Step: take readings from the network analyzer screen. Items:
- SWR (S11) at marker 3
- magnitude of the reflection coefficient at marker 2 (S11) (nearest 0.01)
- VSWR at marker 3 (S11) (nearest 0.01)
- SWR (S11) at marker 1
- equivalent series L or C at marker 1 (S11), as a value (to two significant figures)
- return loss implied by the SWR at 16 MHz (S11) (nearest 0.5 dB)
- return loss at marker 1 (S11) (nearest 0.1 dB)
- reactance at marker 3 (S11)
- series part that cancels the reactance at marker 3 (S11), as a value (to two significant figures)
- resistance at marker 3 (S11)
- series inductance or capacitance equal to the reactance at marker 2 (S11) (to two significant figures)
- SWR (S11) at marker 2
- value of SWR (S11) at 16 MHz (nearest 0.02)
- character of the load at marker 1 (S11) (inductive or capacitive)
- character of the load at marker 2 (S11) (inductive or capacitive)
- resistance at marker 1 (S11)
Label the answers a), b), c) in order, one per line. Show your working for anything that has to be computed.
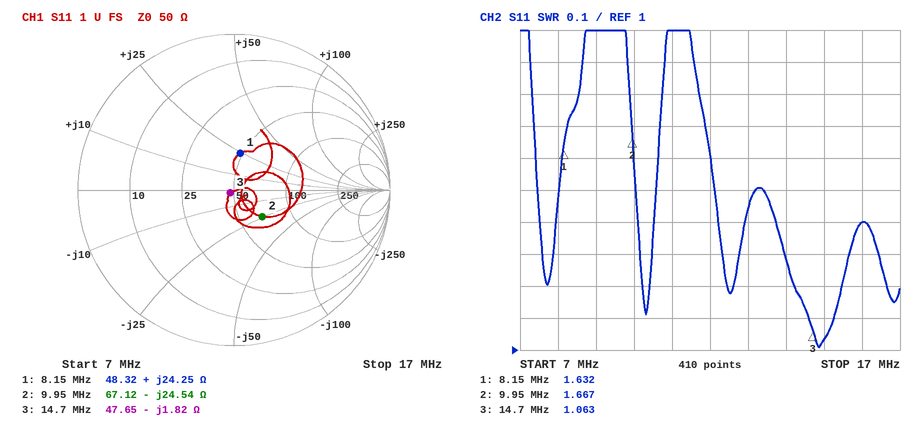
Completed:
a) 1.063
b) 0.25
c) 1.06
d) 1.632
e) L = 24.25 Ω/(2π × 8.15 MHz) ≈ 474 nH, so 470 nH to two significant figures
f) −20 log10((1.4 − 1)/(1.4 + 1)) ≈ 15.6 dB, so 15.5 dB to the nearest 0.5 dB
g) 12.4 dB
h) -1.82 Ω
i) L = 1.82 Ω/(2π × 14.7 MHz) ≈ 20 nH
j) 47.65 Ω
k) C = 1/(2π × 9.95 MHz × 24.54 Ω) ≈ 652 pF, so 650 pF to two significant figures
l) 1.667
m) 1.40
n) inductive
o) capacitive
p) 48.32 Ω
